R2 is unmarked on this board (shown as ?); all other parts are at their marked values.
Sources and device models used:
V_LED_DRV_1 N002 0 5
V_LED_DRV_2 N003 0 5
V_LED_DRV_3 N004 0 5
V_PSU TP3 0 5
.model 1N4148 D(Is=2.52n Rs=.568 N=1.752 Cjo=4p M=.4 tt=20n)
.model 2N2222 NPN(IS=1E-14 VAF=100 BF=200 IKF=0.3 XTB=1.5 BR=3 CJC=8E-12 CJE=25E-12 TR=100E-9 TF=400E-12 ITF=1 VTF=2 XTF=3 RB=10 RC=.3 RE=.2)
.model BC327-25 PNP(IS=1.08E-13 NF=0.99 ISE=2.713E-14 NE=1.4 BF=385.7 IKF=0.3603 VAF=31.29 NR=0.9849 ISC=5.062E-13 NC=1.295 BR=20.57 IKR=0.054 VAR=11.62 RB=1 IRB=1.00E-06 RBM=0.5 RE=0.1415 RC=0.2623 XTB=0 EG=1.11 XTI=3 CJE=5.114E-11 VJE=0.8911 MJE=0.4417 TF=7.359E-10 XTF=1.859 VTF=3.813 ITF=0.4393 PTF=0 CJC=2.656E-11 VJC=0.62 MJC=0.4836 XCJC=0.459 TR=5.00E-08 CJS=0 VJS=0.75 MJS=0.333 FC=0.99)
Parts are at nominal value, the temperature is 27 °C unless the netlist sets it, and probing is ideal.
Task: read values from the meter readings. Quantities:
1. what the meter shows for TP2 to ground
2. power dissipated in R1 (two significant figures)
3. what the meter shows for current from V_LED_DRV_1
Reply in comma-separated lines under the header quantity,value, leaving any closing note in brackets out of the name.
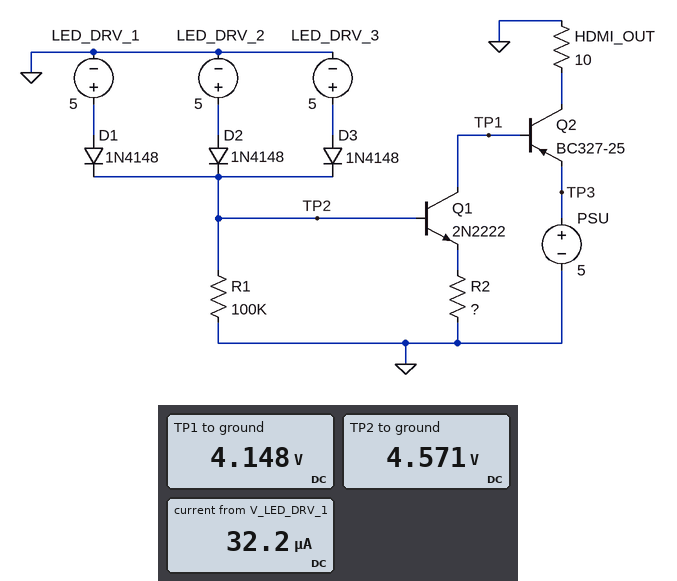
quantity,value
what the meter shows for TP2 to ground,4.571 V
power dissipated in R1,210 µW
what the meter shows for current from V_LED_DRV_1,32.2 µA
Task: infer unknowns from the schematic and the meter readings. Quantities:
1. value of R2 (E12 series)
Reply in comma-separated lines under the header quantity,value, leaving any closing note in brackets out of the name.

quantity,value
value of R2,390 Ω
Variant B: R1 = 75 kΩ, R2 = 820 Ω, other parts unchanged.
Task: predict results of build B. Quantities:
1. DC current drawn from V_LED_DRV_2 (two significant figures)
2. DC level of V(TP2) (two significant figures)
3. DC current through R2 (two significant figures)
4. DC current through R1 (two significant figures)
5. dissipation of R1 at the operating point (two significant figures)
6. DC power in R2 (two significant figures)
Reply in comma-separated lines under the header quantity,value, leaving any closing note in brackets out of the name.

quantity,value
DC current drawn from V_LED_DRV_2,28 µA
DC level of V(TP2),4.6 V
DC current through R2,4.7 mA
DC current through R1,61 µA
dissipation of R1 at the operating point,280 µW
DC power in R2,18 mW
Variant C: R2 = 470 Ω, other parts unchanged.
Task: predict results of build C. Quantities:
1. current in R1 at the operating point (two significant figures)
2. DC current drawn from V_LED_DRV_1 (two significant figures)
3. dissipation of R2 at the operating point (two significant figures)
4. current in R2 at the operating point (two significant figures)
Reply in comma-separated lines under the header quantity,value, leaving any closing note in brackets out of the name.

quantity,value
current in R1 at the operating point,46 µA
DC current drawn from V_LED_DRV_1,29 µA
dissipation of R2 at the operating point,32 mW
current in R2 at the operating point,8.2 mA
